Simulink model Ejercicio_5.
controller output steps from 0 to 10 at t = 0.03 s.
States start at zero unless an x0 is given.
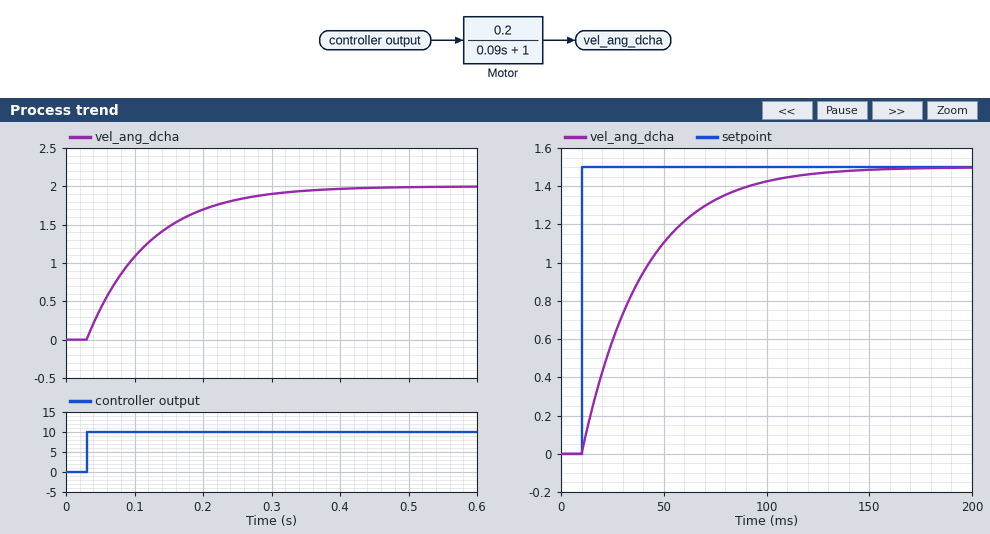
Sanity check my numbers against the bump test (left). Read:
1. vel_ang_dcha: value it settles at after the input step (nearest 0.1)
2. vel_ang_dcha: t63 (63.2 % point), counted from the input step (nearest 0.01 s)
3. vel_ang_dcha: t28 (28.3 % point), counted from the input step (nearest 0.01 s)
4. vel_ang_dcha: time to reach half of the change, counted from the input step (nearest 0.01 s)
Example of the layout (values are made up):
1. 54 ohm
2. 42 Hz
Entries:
1. 2.0
2. 0.09 s
3. 0.03 s
4. 0.06 s
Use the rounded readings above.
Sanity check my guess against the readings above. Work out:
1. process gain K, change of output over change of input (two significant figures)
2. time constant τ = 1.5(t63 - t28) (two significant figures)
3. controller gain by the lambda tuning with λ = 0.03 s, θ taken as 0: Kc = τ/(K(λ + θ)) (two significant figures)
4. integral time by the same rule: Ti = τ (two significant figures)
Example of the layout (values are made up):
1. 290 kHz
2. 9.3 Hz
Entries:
1. 0.20
2. 0.090 s
3. 15
4. 0.090 s
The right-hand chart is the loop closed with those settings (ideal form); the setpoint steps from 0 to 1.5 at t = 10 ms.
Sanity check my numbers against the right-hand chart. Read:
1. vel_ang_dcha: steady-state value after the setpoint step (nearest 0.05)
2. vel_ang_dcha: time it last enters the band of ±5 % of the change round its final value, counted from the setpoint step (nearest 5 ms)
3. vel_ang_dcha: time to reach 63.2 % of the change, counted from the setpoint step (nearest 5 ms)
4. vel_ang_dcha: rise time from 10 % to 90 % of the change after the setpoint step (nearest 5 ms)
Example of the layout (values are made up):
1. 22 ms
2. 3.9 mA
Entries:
1. 1.50
2. 90 ms
3. 30 ms
4. 65 ms
